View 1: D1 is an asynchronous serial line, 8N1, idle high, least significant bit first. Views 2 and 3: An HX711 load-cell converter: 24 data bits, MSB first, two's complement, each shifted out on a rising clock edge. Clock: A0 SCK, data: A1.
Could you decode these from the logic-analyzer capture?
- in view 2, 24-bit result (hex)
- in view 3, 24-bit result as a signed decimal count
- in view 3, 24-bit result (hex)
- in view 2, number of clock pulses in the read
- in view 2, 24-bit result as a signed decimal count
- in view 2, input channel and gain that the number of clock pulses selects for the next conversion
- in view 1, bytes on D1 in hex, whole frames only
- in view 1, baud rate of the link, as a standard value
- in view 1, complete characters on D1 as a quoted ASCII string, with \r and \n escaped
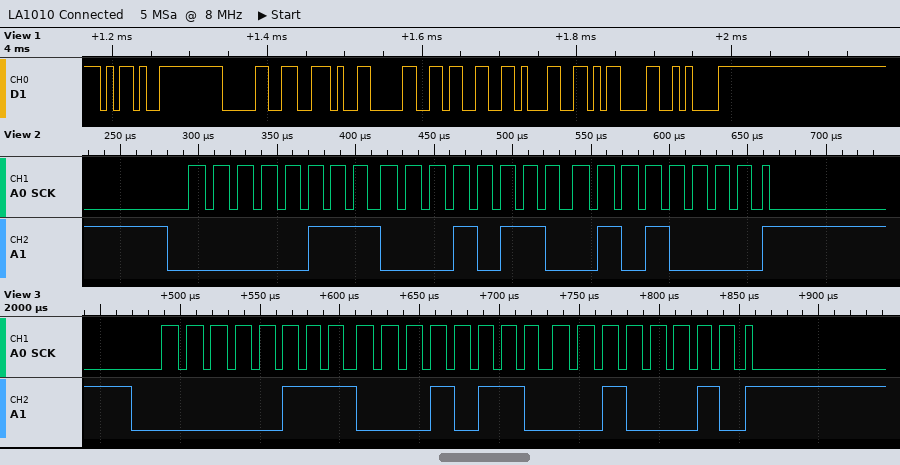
0x071650
464418
0x071622
25
464464
channel A, gain 128
0x2D 0x30 0x2E 0x30 0x33 0x31 0x0D 0x0A
115200 baud
"-0.031\r\n"
